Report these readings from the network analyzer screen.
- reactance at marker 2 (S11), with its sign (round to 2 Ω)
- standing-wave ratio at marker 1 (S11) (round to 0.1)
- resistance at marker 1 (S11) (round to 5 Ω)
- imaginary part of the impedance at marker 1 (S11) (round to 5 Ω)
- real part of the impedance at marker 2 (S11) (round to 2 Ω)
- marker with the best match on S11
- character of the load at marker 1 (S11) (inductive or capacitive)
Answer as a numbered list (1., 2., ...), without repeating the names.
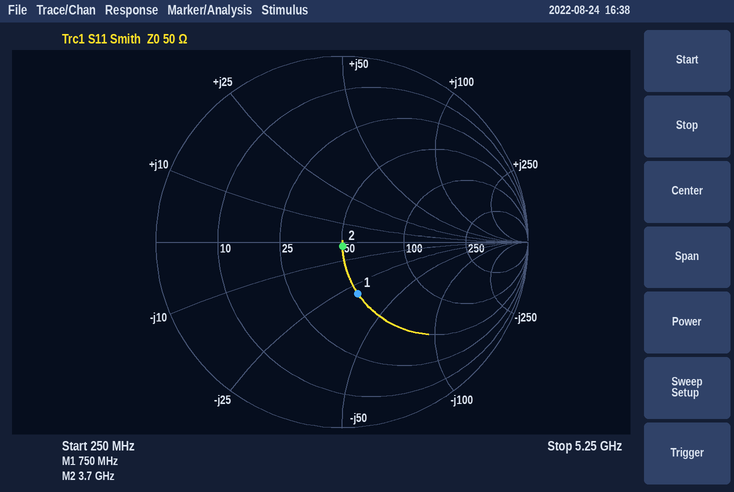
1. -2 Ω
2. 1.8
3. 50 Ω
4. -30 Ω
5. 50 Ω
6. marker 2
7. capacitive
